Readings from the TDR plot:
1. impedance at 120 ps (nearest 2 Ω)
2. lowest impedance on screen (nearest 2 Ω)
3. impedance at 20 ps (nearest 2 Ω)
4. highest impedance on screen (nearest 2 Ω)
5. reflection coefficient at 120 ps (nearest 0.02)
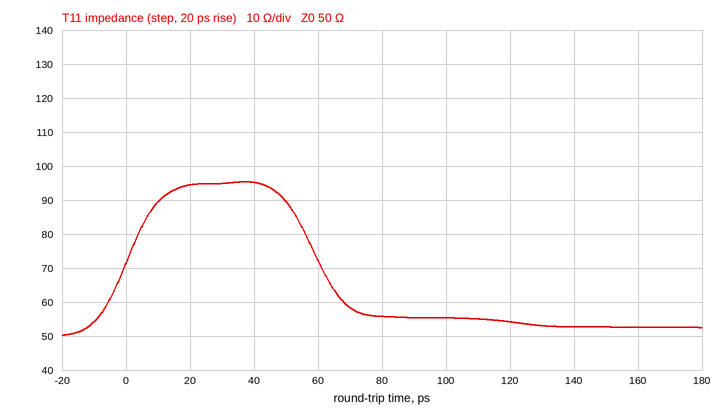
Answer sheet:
54 Ω
50 Ω
94 Ω
96 Ω
+0.04
